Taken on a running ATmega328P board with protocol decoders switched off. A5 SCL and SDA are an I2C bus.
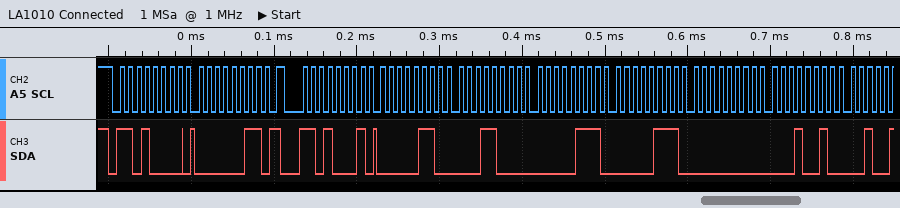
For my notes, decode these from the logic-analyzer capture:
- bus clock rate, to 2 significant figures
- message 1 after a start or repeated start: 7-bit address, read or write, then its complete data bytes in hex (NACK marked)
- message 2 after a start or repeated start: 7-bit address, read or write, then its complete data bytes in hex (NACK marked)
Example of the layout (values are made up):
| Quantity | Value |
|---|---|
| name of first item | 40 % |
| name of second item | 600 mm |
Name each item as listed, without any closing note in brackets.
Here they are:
| Quantity | Value |
|---|---|
| bus clock rate, to 2 significant figures | 100 kHz |
| message 1 after a start or repeated start: 7-bit address, read or write, then its complete data bytes in hex | 0x68 write: 03 |
| message 2 after a start or repeated start: 7-bit address, read or write, then its complete data bytes in hex | 0x68 read: 06 18 07 07 00 12 |
